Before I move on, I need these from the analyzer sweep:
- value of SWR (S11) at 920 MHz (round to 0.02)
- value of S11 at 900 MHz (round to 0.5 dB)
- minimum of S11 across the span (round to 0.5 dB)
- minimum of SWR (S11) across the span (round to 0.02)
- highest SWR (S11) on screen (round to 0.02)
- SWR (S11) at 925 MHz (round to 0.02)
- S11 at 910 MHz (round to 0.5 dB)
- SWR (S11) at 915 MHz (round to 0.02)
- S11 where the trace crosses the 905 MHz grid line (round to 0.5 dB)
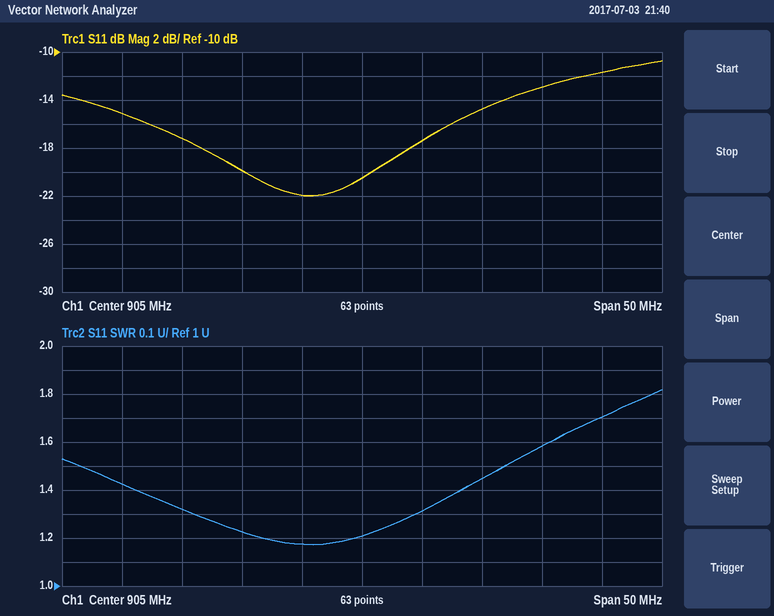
1.58
-22.0 dB
-22.0 dB
1.18
1.82
1.70
-17.5 dB
1.44
-20.5 dB
